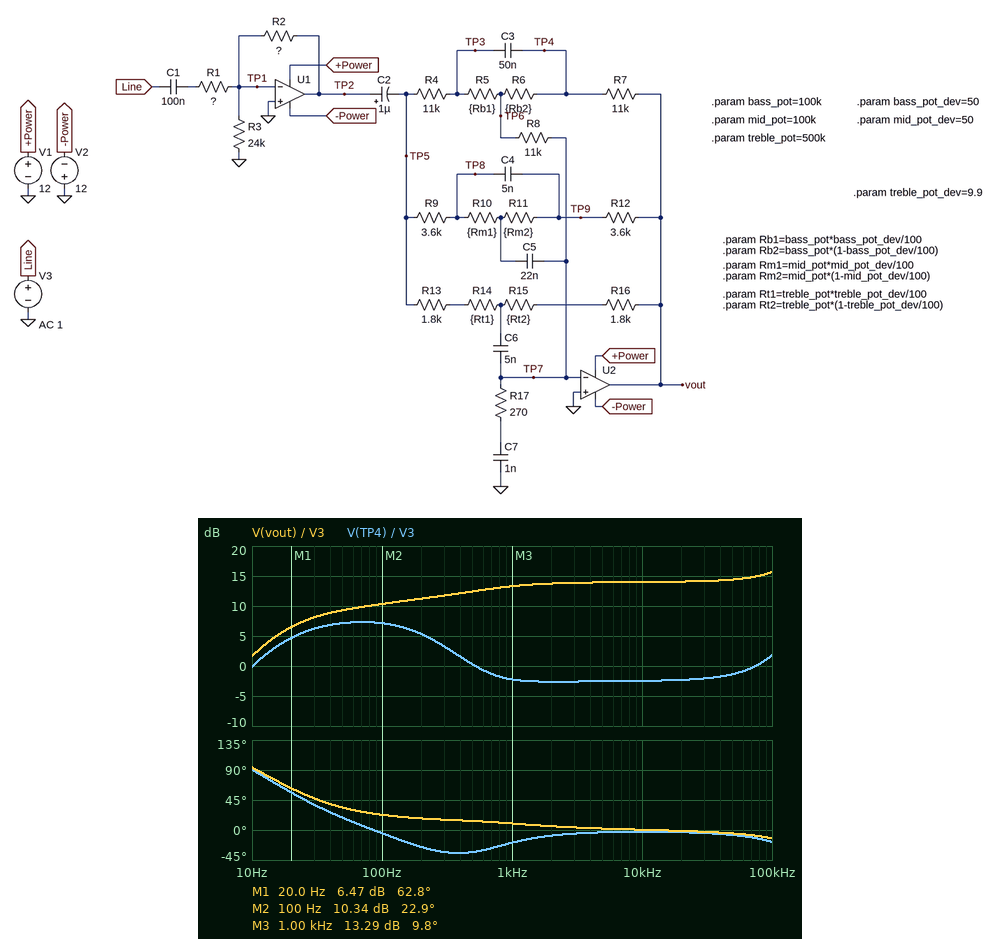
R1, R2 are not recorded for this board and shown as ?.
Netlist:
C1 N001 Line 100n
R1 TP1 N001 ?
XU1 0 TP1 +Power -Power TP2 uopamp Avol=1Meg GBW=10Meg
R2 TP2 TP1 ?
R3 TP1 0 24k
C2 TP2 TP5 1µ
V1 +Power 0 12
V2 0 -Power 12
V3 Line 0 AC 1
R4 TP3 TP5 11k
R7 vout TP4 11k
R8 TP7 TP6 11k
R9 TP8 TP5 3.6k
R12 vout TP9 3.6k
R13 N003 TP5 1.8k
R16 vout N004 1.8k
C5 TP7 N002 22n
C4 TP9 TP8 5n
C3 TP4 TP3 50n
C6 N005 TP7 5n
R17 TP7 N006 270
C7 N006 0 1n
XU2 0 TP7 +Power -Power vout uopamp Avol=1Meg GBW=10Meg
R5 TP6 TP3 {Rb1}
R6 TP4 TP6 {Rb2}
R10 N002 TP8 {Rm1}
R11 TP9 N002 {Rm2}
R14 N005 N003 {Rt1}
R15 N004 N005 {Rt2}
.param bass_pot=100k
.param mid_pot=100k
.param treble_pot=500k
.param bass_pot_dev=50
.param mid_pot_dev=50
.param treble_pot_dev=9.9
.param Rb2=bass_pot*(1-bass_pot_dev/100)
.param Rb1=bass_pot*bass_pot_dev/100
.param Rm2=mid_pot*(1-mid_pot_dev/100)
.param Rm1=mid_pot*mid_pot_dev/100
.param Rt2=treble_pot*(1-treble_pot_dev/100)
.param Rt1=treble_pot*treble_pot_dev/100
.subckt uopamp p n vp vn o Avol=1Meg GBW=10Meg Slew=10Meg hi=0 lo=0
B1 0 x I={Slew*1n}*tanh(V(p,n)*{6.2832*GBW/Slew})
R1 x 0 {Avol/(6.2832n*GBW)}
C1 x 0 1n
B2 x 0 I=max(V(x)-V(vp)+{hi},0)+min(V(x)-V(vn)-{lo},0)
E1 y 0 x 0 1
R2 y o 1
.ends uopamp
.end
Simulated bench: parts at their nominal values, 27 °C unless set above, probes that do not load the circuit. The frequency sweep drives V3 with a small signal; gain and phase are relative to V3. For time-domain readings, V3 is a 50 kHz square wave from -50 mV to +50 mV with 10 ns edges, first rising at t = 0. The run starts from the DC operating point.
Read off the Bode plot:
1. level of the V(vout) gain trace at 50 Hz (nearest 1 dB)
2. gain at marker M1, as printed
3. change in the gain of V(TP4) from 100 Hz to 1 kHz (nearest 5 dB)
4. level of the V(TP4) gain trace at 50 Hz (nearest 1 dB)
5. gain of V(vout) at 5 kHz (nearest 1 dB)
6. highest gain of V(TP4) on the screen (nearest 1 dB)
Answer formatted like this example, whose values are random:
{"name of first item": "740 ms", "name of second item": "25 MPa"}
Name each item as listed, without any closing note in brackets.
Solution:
{"level of the V(vout) gain trace at 50 Hz": "9 dB", "gain at marker M1, as printed": "6.47 dB", "change in the gain of V(TP4) from 100 Hz to 1 kHz": "-10 dB", "level of the V(TP4) gain trace at 50 Hz": "7 dB", "gain of V(vout) at 5 kHz": "14 dB", "highest gain of V(TP4) on the screen": "7 dB"}
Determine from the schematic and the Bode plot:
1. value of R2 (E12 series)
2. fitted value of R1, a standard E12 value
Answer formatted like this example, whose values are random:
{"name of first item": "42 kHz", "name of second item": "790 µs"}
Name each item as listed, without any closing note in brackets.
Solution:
{"value of R2": "270 kΩ", "fitted value of R1, a standard E12 value": "82 kΩ"}
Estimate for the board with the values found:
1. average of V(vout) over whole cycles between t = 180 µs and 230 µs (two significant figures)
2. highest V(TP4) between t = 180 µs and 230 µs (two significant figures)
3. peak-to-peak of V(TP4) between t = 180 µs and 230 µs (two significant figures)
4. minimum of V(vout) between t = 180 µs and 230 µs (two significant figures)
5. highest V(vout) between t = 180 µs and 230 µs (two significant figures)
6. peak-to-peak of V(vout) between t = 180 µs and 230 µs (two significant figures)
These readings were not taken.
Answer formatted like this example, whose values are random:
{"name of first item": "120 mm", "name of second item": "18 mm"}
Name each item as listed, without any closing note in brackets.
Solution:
{"average of V(vout) over whole cycles between t = 180 µs and 230 µs": "200 mV", "highest V(TP4) between t = 180 µs and 230 µs": "200 mV", "peak-to-peak of V(TP4) between t = 180 µs and 230 µs": "290 mV", "minimum of V(vout) between t = 180 µs and 230 µs": "-300 mV", "highest V(vout) between t = 180 µs and 230 µs": "700 mV", "peak-to-peak of V(vout) between t = 180 µs and 230 µs": "1.0 V"}
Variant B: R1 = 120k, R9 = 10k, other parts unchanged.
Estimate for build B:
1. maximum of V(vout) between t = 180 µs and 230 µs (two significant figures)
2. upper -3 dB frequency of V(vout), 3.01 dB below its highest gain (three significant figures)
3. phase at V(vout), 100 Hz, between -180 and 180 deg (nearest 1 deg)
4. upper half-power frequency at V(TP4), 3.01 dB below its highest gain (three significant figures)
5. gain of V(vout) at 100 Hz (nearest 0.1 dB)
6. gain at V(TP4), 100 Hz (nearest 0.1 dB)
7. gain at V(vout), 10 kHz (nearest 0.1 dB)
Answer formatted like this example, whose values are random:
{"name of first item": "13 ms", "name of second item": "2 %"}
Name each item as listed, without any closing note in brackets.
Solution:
{"maximum of V(vout) between t = 180 µs and 230 µs": "350 mV", "upper -3 dB frequency of V(vout), 3.01 dB below its highest gain": "294 kHz", "phase at V(vout), 100 Hz, between -180 and 180 deg": "17 deg", "upper half-power frequency at V(TP4), 3.01 dB below its highest gain": "367 kHz", "gain of V(vout) at 100 Hz": "6.9 dB", "gain at V(TP4), 100 Hz": "3.8 dB", "gain at V(vout), 10 kHz": "7.3 dB"}
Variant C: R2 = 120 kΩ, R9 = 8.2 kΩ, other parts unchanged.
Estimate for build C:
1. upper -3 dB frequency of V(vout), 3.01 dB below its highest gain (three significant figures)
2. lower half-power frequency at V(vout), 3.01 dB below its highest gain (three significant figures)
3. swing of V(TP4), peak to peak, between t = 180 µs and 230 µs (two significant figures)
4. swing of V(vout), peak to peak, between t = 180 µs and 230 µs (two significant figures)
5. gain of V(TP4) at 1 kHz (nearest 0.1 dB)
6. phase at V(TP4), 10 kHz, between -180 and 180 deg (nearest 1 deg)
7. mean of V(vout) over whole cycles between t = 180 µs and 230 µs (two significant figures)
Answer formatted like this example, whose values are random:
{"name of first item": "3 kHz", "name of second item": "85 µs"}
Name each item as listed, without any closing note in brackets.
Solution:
{"upper -3 dB frequency of V(vout), 3.01 dB below its highest gain": "291 kHz", "lower half-power frequency at V(vout), 3.01 dB below its highest gain": "167 kHz", "swing of V(TP4), peak to peak, between t = 180 µs and 230 µs": "110 mV", "swing of V(vout), peak to peak, between t = 180 µs and 230 µs": "320 mV", "gain of V(TP4) at 1 kHz": "-9.6 dB", "phase at V(TP4), 10 kHz, between -180 and 180 deg": "-48 deg", "mean of V(vout) over whole cycles between t = 180 µs and 230 µs": "87 mV"}
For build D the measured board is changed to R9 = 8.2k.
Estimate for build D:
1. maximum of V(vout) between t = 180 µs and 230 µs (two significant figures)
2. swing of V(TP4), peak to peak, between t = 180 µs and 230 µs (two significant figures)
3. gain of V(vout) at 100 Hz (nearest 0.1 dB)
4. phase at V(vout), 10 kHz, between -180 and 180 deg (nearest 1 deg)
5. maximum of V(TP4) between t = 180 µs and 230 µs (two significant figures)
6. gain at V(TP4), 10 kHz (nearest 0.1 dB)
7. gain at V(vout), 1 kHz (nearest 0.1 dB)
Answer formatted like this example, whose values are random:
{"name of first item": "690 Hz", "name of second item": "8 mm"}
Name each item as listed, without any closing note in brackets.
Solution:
{"maximum of V(vout) between t = 180 µs and 230 µs": "540 mV", "swing of V(TP4), peak to peak, between t = 180 µs and 230 µs": "200 mV", "gain of V(vout) at 100 Hz": "10.2 dB", "phase at V(vout), 10 kHz, between -180 and 180 deg": "-5 deg", "maximum of V(TP4) between t = 180 µs and 230 µs": "150 mV", "gain at V(TP4), 10 kHz": "-13.1 dB", "gain at V(vout), 1 kHz": "12.8 dB"}
